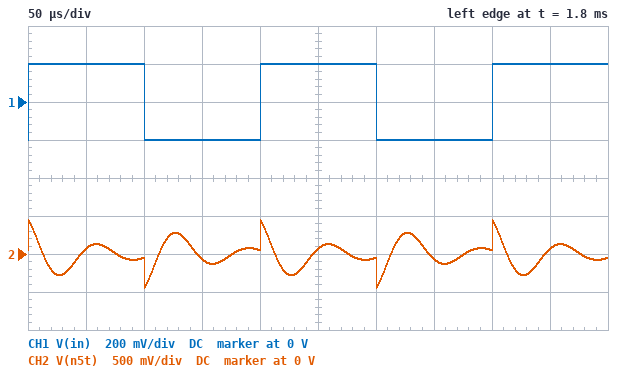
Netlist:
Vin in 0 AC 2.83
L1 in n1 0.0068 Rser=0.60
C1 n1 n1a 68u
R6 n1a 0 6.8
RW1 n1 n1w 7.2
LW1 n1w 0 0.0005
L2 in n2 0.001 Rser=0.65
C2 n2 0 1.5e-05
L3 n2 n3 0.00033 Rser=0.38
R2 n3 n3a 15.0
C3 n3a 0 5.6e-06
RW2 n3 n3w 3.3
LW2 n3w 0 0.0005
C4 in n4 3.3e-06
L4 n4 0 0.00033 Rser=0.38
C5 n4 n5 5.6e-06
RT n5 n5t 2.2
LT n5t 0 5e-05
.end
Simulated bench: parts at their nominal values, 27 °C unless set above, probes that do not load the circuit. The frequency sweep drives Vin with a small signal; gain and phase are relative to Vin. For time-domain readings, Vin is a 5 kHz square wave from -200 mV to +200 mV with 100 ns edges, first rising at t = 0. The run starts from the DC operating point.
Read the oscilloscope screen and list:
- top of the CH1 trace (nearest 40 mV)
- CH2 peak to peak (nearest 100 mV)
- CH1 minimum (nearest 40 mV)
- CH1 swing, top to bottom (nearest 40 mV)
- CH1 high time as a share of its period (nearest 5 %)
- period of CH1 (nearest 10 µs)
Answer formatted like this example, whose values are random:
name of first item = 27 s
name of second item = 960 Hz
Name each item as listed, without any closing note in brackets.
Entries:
top of the CH1 trace = 200 mV
CH2 peak to peak = 900 mV
CH1 minimum = -200 mV
CH1 swing, top to bottom = 400 mV
CH1 high time as a share of its period = 50 %
period of CH1 = 200 µs
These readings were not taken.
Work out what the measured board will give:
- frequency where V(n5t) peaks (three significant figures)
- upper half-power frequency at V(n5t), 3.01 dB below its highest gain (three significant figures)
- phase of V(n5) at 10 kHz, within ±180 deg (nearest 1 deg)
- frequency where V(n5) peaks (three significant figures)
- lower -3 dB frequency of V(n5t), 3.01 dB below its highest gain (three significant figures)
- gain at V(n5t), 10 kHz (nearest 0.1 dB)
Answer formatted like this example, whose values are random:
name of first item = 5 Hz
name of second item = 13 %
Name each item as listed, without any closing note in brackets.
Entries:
frequency where V(n5t) peaks = 16.7 kHz
upper half-power frequency at V(n5t), 3.01 dB below its highest gain = 22.1 kHz
phase of V(n5) at 10 kHz, within ±180 deg = 125 deg
frequency where V(n5) peaks = 16.6 kHz
lower -3 dB frequency of V(n5t), 3.01 dB below its highest gain = 13.9 kHz
gain at V(n5t), 10 kHz = -3.9 dB
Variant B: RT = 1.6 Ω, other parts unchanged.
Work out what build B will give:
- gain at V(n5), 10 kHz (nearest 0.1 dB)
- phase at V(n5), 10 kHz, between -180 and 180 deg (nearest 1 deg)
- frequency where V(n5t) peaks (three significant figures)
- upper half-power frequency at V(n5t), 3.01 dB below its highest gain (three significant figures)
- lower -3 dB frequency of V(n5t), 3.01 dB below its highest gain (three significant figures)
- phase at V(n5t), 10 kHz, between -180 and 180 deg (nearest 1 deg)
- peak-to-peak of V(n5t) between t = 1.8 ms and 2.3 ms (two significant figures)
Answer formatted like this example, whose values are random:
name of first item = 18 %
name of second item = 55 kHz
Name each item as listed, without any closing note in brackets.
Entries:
gain at V(n5), 10 kHz = -2.6 dB
phase at V(n5), 10 kHz, between -180 and 180 deg = 138 deg
frequency where V(n5t) peaks = 16.4 kHz
upper half-power frequency at V(n5t), 3.01 dB below its highest gain = 19.7 kHz
lower -3 dB frequency of V(n5t), 3.01 dB below its highest gain = 14.3 kHz
phase at V(n5t), 10 kHz, between -180 and 180 deg = 165 deg
peak-to-peak of V(n5t) between t = 1.8 ms and 2.3 ms = 960 mV
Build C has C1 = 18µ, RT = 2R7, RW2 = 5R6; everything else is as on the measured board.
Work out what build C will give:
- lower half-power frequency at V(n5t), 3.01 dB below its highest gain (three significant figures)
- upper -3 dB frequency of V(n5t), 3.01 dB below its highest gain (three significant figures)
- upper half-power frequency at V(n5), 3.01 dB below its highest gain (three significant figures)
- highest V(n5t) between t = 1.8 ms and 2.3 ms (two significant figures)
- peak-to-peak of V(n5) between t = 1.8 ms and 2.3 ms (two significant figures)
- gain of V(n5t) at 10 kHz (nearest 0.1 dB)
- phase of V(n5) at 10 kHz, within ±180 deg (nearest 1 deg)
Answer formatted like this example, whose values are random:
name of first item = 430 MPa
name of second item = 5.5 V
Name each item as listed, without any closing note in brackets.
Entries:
lower half-power frequency at V(n5t), 3.01 dB below its highest gain = 13.6 kHz
upper -3 dB frequency of V(n5t), 3.01 dB below its highest gain = 25.3 kHz
upper half-power frequency at V(n5), 3.01 dB below its highest gain = 23.8 kHz
highest V(n5t) between t = 1.8 ms and 2.3 ms = 430 mV
peak-to-peak of V(n5) between t = 1.8 ms and 2.3 ms = 930 mV
gain of V(n5t) at 10 kHz = -4.1 dB
phase of V(n5) at 10 kHz, within ±180 deg = 115 deg
